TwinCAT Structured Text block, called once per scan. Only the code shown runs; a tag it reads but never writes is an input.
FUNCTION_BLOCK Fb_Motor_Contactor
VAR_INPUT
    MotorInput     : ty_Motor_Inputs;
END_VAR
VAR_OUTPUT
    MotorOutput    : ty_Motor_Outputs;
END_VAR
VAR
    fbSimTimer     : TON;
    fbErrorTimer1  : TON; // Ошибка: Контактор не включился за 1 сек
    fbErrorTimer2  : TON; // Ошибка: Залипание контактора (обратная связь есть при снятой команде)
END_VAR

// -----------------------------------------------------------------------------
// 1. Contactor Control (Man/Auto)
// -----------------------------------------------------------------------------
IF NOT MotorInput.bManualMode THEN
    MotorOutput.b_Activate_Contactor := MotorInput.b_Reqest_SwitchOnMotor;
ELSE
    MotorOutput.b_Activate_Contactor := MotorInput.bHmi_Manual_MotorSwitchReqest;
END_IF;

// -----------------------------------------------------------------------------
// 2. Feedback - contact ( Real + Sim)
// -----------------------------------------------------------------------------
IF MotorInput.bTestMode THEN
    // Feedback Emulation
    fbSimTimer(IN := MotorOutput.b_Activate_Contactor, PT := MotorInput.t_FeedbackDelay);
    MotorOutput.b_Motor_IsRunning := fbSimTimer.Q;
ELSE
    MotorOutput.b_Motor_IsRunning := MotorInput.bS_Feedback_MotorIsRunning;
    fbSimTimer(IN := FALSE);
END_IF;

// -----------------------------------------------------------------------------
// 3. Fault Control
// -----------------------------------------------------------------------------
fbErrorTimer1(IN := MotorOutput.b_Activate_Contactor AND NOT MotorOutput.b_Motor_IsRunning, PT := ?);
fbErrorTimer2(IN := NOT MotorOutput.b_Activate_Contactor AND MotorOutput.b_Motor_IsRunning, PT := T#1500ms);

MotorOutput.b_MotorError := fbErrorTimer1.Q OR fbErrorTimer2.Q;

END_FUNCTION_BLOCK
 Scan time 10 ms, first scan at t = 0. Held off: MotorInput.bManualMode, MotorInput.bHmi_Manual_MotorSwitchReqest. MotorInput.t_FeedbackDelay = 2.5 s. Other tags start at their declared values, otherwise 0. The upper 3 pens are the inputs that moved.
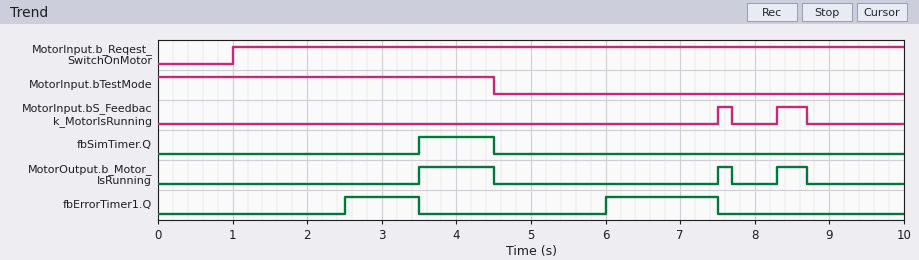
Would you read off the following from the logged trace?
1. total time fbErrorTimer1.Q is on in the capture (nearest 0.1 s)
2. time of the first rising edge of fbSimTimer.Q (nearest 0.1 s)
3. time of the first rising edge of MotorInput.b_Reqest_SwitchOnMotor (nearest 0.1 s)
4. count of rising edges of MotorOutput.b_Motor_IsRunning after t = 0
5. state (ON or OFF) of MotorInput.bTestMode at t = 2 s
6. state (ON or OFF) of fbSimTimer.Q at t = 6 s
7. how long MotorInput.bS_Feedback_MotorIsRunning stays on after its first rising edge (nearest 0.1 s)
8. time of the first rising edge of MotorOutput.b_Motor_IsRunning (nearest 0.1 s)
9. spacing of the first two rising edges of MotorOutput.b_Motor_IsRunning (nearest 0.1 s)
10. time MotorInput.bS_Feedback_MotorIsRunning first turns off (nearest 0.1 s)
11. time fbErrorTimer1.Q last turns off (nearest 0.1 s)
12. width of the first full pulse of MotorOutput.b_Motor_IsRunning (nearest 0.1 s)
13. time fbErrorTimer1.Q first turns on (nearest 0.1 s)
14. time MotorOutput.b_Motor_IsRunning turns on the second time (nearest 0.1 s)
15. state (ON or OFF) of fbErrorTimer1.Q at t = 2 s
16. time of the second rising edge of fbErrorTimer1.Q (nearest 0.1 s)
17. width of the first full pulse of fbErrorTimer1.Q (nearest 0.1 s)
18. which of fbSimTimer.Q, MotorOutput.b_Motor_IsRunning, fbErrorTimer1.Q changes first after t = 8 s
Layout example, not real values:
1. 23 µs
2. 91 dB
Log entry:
1. 2.5 s
2. 3.5 s
3. 1.0 s
4. 3
5. ON
6. OFF
7. 0.2 s
8. 3.5 s
9. 4.0 s
10. 7.7 s
11. 7.5 s
12. 1.0 s
13. 2.5 s
14. 7.5 s
15. OFF
16. 6.0 s
17. 1.0 s
18. MotorOutput.b_Motor_IsRunning
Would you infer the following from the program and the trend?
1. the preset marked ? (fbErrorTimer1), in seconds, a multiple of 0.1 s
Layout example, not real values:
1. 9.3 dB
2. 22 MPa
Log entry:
1. 1.5 s
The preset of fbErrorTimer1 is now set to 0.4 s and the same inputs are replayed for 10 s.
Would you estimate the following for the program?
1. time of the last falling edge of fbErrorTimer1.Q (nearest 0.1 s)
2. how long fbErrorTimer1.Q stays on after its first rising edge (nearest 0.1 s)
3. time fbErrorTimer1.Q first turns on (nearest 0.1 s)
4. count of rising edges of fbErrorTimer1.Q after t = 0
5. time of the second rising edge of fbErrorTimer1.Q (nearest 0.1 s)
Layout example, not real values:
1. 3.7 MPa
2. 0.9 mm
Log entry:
1. 8.3 s
2. 2.1 s
3. 1.4 s
4. 4
5. 4.9 s
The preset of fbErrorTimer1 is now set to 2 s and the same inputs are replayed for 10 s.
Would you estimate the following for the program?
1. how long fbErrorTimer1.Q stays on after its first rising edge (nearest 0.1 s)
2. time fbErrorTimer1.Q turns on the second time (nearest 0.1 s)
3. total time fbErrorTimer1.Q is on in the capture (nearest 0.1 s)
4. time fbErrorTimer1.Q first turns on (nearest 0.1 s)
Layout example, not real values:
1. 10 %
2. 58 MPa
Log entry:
1. 0.5 s
2. 6.5 s
3. 1.5 s
4. 3.0 s
